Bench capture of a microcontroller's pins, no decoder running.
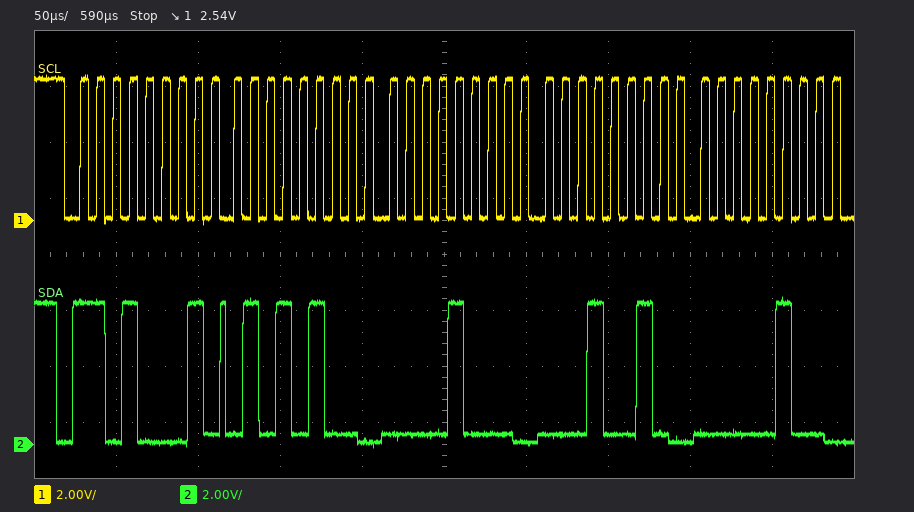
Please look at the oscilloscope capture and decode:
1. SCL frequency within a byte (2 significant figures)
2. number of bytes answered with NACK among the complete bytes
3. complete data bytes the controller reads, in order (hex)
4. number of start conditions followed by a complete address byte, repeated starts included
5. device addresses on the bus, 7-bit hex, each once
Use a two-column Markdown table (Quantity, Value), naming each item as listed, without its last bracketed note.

| Quantity | Value |
|---|---|
| SCL frequency within a byte | 100 kHz |
| number of bytes answered with NACK among the complete bytes | 0 |
| complete data bytes the controller reads, in order | 54 08 12 04 |
| number of start conditions followed by a complete address byte, repeated starts included | 1 |
| device addresses on the bus, 7-bit hex, each once | 0x68 |
